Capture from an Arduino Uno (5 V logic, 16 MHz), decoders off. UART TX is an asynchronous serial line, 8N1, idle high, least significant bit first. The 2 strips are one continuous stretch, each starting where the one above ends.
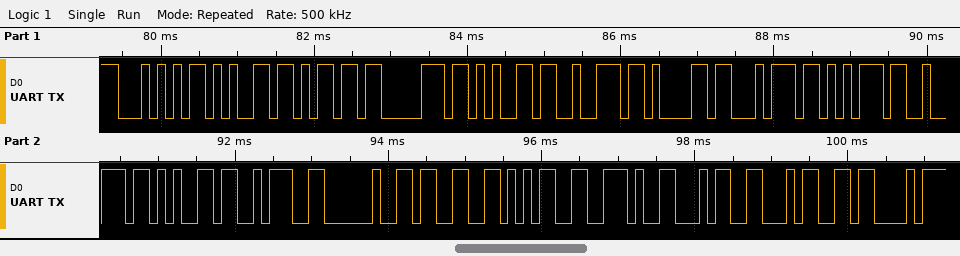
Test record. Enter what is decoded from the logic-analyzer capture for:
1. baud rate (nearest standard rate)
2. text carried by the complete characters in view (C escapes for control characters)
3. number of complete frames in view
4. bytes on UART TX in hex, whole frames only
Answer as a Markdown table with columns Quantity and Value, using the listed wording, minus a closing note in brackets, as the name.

| Quantity | Value |
|---|---|
| baud rate | 9600 baud |
| text carried by the complete characters in view | "Temperature: 35.44C" |
| number of complete frames in view | 19 |
| bytes on UART TX in hex, whole frames only | 0x54 0x65 0x6D 0x70 0x65 0x72 0x61 0x74 0x75 0x72 0x65 0x3A 0x20 0x33 0x35 0x2E 0x34 0x34 0x43 |
